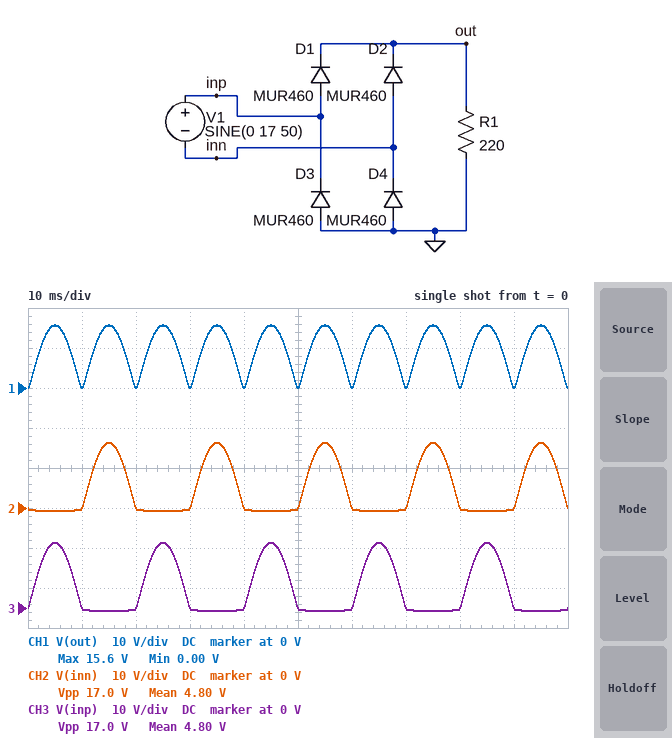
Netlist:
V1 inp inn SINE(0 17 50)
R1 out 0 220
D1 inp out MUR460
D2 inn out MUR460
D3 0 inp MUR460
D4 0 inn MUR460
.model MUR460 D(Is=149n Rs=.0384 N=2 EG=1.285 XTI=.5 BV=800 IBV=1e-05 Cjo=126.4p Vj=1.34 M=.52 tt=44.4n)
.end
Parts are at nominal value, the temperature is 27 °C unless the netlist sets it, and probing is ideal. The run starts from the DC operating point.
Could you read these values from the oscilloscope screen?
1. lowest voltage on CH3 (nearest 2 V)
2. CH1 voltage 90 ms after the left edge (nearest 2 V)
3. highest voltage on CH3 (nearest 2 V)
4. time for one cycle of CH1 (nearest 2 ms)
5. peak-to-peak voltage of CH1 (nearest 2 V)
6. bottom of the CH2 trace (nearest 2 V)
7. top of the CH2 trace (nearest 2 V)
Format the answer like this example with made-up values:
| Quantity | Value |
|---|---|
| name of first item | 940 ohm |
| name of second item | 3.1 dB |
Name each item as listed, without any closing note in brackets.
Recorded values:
| Quantity | Value |
|---|---|
| lowest voltage on CH3 | 0 V |
| CH1 voltage 90 ms after the left edge | 0 V |
| highest voltage on CH3 | 16 V |
| time for one cycle of CH1 | 10 ms |
| peak-to-peak voltage of CH1 | 16 V |
| bottom of the CH2 trace | 0 V |
| top of the CH2 trace | 16 V |
